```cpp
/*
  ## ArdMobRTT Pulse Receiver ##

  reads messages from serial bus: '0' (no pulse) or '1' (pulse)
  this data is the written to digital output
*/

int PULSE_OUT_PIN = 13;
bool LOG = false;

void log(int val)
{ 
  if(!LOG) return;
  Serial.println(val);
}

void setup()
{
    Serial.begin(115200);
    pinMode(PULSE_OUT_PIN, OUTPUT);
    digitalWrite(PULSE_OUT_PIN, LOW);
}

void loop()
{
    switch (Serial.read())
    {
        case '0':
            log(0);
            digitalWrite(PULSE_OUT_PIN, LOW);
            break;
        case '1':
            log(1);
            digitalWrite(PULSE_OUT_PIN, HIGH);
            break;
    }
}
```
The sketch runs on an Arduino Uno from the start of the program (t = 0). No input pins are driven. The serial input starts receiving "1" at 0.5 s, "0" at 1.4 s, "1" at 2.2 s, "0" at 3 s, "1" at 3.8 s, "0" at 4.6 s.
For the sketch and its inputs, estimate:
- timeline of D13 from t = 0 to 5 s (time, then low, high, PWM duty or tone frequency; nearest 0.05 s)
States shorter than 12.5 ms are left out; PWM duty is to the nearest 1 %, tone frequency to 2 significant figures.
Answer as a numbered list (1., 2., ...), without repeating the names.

1. 0 s low; 0.5 s high; 1.4 s low; 2.2 s high; 3 s low; 3.8 s high; 4.6 s low
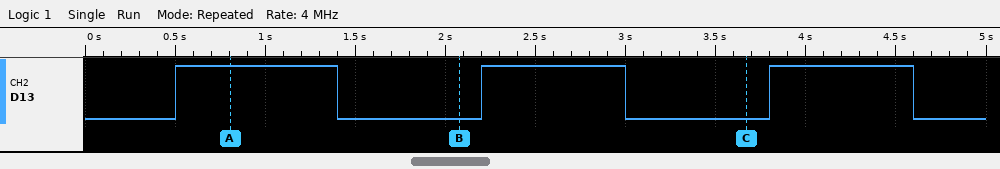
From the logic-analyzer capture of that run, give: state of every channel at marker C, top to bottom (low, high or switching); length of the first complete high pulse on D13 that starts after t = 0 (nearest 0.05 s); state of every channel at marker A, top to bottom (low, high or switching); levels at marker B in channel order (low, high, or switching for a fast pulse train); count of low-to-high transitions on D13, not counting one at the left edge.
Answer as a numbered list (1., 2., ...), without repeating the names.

1. D13 low
2. 0.90 s
3. D13 high
4. D13 low
5. 3
